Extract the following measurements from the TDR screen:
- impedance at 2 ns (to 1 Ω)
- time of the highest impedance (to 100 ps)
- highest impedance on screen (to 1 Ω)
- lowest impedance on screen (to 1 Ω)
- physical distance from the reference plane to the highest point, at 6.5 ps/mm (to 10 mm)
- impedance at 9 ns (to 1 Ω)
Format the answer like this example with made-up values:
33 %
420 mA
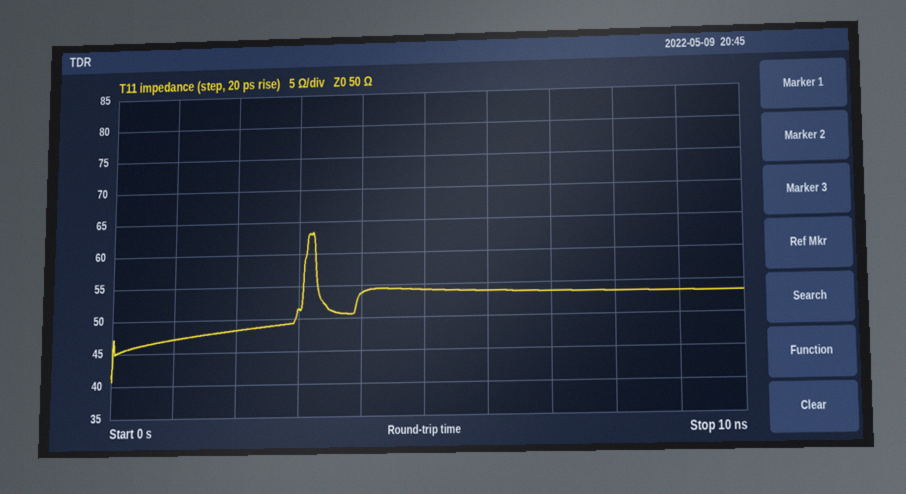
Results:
48 Ω
3.2 ns
63 Ω
41 Ω
250 mm
53 Ω
